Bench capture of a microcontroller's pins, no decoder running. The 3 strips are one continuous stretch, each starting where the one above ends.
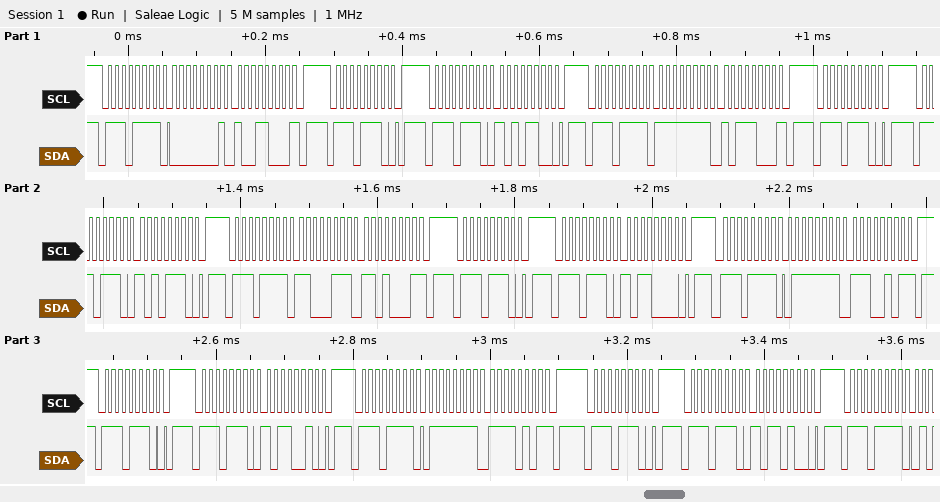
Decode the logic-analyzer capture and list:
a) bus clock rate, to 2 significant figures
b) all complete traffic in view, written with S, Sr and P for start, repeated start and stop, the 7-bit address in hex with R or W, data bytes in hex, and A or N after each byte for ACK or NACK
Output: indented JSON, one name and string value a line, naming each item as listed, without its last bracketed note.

{
  "bus clock rate, to 2 significant figures": "100 kHz",
  "all complete traffic in view, written with S, Sr and P for start, repeated start and stop, the 7-bit address in hex with R or W, data bytes in hex, and A or N after each byte for ACK or NACK": "S 77R A 01 A 98 N P S 77W A P S 77W A AC A P S 77R A FF A B8 N P S 77W A P S 77W A AE A P S 77R A C7 A D1 N P S 77W A P S 77W A B0 A P S 77R A 7F A E5 N P S 77W A P S 77W A B2 A P S 77R A 7F A F5 N P S 77W A P S 77W A B4 A P S 77R A"
}
